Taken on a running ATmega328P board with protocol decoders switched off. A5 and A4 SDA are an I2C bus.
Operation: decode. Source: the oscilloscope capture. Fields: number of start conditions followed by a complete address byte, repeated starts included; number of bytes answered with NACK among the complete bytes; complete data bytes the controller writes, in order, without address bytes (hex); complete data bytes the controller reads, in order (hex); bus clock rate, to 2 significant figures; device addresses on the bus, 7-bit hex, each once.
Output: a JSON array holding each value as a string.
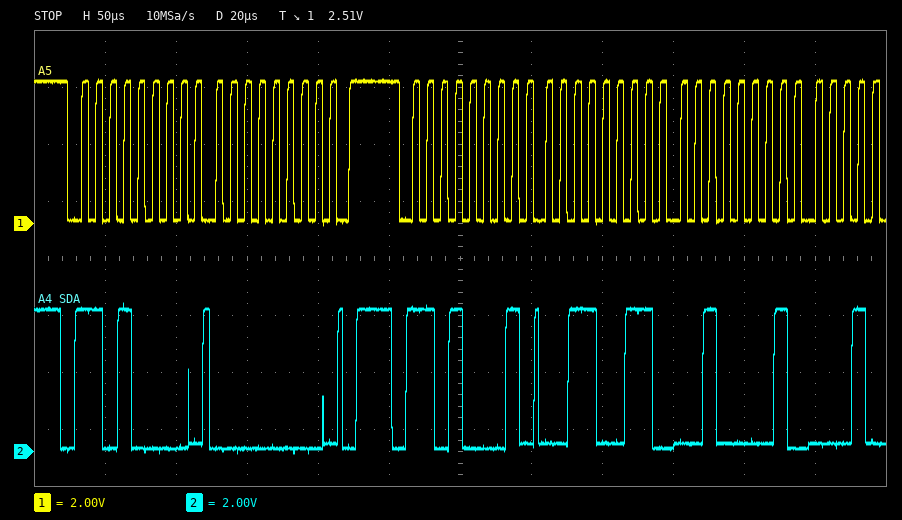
["2", "0", "00", "33 21", "100 kHz", "0x68"]
